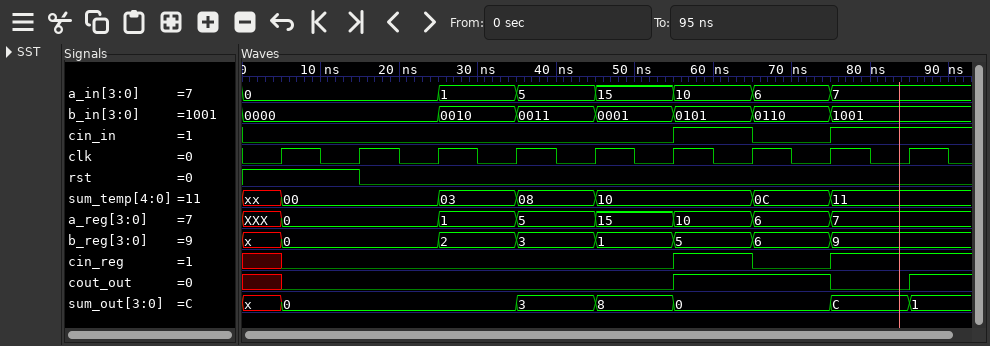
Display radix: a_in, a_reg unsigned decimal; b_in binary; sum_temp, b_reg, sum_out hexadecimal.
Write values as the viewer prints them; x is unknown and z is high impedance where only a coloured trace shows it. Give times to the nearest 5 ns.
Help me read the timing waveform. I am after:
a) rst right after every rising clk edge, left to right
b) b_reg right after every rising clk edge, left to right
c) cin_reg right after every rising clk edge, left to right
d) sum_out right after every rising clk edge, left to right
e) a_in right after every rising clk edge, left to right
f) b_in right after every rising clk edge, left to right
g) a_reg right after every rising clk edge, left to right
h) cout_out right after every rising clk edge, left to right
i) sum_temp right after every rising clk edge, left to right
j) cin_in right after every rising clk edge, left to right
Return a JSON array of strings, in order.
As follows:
["1 0 0 0 0 0 0 0 0", "0, 0, 2, 3, 1, 5, 6, 9, 9", "0 0 0 0 0 1 0 1 1", "0, 0, 0, 3, 8, 0, 0, C, 1", "0, 0, 1, 5, 15, 10, 6, 7, 7", "0000, 0000, 0010, 0011, 0001, 0101, 0110, 1001, 1001", "0, 0, 1, 5, 15, 10, 6, 7, 7", "0 0 0 0 0 1 1 0 1", "00, 00, 03, 08, 10, 10, 0C, 11, 11", "0 0 0 0 0 1 0 1 1"]
